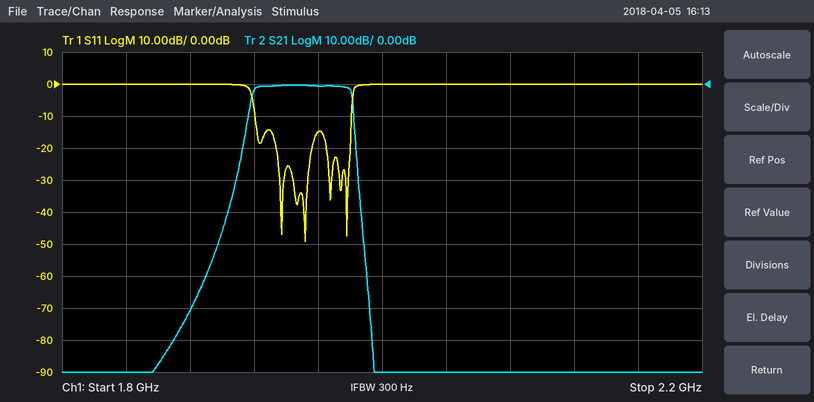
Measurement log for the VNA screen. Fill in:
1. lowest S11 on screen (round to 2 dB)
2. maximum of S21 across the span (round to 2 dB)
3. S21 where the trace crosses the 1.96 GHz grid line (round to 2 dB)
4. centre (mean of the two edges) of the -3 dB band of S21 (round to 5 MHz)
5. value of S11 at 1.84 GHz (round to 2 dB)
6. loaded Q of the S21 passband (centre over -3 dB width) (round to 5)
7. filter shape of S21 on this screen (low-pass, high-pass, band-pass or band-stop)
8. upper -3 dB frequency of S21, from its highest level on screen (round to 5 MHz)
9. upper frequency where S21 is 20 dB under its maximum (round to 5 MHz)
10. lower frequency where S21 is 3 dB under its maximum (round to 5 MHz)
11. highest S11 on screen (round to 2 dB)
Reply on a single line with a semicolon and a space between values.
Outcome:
-50 dB; 0 dB; 0 dB; 1.950 GHz; 0 dB; 30; band-pass; 1.980 GHz; 1.985 GHz; 1.920 GHz; 0 dB
